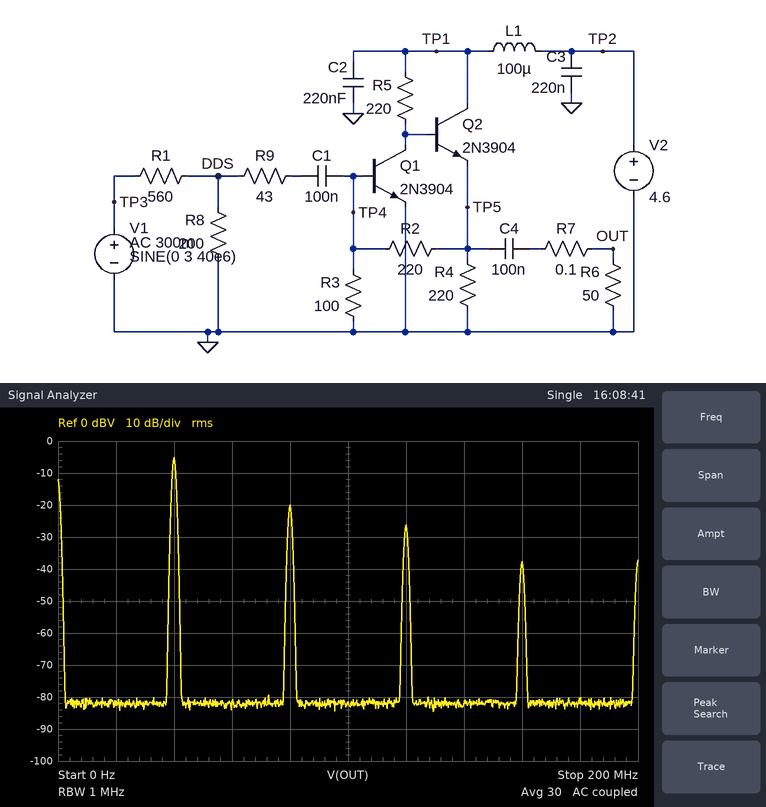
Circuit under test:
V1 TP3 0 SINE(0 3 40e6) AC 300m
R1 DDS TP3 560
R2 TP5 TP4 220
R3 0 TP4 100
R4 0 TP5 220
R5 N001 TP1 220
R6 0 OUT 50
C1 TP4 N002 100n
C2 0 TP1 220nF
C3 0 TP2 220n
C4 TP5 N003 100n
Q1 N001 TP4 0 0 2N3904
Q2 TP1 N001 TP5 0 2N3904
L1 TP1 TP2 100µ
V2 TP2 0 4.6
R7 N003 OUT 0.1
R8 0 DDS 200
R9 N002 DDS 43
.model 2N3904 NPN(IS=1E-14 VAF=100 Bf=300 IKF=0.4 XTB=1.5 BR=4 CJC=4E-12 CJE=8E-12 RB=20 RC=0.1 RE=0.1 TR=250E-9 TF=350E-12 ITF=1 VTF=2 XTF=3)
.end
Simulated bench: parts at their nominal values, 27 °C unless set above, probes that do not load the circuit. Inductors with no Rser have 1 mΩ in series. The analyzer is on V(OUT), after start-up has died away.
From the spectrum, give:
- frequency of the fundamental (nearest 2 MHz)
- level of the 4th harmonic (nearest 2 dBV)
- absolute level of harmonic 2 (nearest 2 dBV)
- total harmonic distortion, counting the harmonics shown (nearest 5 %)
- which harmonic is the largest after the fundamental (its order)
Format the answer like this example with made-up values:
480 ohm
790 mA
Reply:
40 MHz
-38 dBV
-20 dBV
20 %
2
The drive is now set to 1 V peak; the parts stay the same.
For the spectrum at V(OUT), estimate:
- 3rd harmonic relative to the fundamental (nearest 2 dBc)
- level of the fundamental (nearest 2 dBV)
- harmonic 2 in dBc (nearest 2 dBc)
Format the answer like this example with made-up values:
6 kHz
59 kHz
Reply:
-54 dBc
-14 dBV
-56 dBc
